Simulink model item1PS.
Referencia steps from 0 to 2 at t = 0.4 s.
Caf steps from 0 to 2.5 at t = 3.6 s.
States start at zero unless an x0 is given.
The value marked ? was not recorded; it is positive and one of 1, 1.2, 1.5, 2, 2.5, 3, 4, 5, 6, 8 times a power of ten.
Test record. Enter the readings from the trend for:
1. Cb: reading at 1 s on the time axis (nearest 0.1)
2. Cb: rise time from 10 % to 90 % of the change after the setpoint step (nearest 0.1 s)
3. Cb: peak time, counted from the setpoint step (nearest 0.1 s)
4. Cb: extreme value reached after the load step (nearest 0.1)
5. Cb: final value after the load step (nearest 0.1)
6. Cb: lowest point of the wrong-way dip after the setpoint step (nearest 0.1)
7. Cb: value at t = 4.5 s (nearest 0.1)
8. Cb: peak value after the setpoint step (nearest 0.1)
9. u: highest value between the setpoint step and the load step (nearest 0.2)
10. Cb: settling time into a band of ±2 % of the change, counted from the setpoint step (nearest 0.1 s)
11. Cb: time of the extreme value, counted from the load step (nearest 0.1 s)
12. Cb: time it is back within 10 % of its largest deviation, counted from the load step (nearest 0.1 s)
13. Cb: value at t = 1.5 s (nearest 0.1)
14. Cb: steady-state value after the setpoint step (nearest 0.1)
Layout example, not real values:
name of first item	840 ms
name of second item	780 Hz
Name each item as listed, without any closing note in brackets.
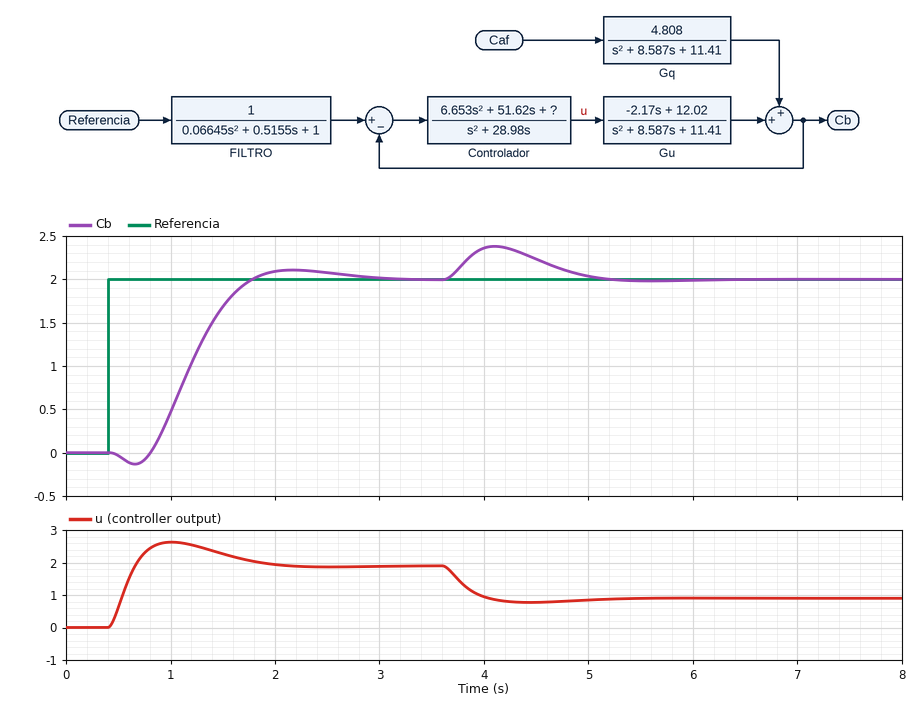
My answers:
Cb: reading at 1 s on the time axis	0.5
Cb: rise time from 10 % to 90 % of the change after the setpoint step	0.7 s
Cb: peak time, counted from the setpoint step	1.8 s
Cb: extreme value reached after the load step	2.4
Cb: final value after the load step	2.0
Cb: lowest point of the wrong-way dip after the setpoint step	-0.1
Cb: value at t = 4.5 s	2.2
Cb: peak value after the setpoint step	2.1
u: highest value between the setpoint step and the load step	2.6
Cb: settling time into a band of ±2 % of the change, counted from the setpoint step	2.4 s
Cb: time of the extreme value, counted from the load step	0.5 s
Cb: time it is back within 10 % of its largest deviation, counted from the load step	1.4 s
Cb: value at t = 1.5 s	1.7
Cb: steady-state value after the setpoint step	2.0
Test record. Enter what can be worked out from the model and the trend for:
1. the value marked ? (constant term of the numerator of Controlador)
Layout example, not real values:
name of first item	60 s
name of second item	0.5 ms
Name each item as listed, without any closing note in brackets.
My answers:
the value marked ?	100
